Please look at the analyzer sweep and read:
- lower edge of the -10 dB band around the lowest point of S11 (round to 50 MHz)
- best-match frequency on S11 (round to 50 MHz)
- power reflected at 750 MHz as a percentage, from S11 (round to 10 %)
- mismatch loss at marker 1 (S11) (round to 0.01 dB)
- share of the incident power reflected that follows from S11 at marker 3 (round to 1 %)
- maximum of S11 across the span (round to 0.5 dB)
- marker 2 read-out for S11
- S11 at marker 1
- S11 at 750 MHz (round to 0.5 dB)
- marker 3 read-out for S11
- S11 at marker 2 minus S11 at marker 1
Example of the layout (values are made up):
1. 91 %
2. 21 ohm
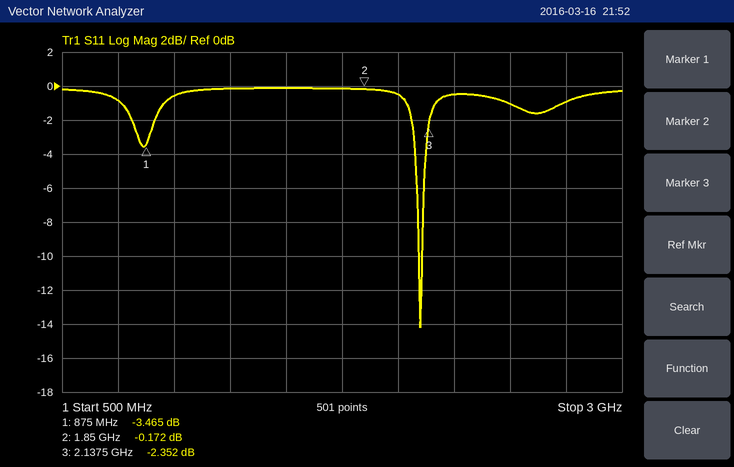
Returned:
1. 2.10 GHz
2. 2.10 GHz
3. 80 %
4. 2.60 dB
5. 58 %
6. 0.0 dB
7. -0.172 dB
8. -3.465 dB
9. -1.0 dB
10. -2.352 dB
11. 3.293 dB
